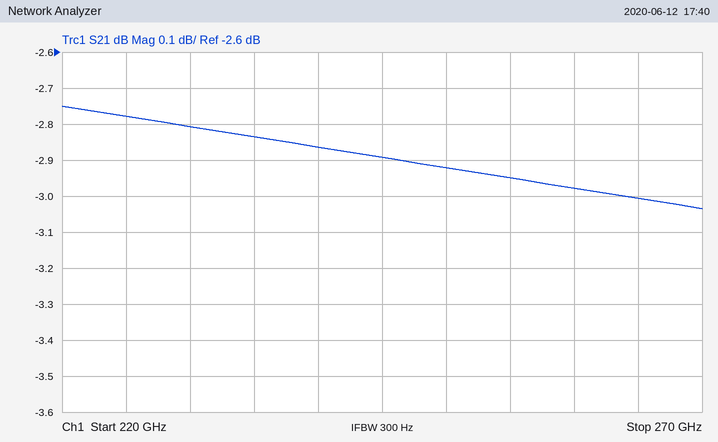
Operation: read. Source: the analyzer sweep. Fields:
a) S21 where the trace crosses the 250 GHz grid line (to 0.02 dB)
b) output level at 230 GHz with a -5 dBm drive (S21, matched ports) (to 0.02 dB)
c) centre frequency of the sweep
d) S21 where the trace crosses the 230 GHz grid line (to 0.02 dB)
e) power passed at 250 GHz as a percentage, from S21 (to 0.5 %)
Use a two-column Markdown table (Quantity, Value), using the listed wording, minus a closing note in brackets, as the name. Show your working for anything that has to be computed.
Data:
| Quantity | Value |
|---|---|
| S21 where the trace crosses the 250 GHz grid line | -2.92 dB |
| output level at 230 GHz with a -5 dBm drive (S21, matched ports) | -5 dBm + (-2.80 dB) = -7.80 dBm |
| centre frequency of the sweep | 245 GHz |
| S21 where the trace crosses the 230 GHz grid line | -2.80 dB |
| power passed at 250 GHz as a percentage, from S21 | 10^(-2.92/10) ≈ 51.1 %, so 51.0 % to the nearest 0.5 % |
